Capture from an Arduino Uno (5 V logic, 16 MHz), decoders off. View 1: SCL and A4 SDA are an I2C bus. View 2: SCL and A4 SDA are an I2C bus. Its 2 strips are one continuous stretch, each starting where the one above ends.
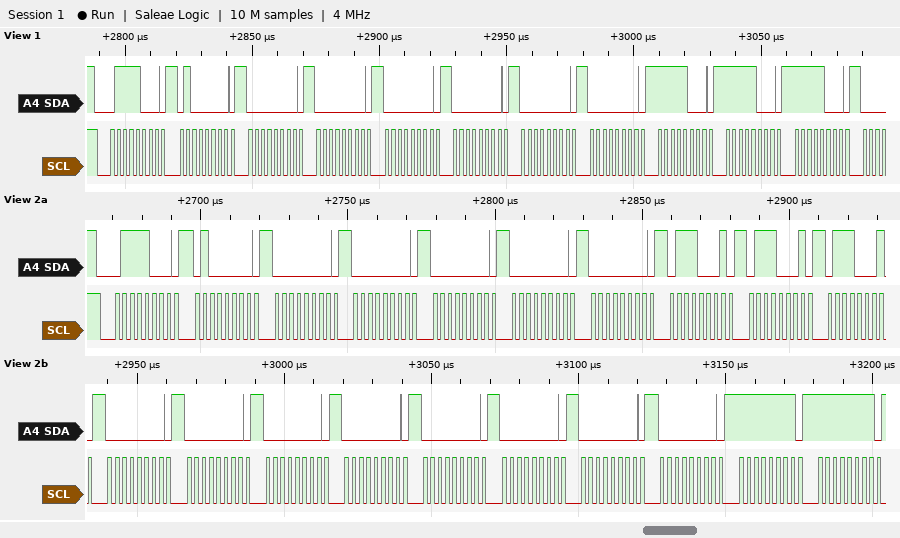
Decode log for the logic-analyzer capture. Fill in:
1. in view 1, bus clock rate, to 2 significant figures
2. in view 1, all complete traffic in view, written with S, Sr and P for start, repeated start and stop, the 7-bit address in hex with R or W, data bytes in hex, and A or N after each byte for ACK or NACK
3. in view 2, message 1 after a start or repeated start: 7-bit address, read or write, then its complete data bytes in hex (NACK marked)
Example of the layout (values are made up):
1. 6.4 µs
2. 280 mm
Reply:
1. 400 kHz
2. S 3CW A 40 A 00 A 00 A 00 A 00 A 00 A 00 A F8 A F8 A F8 A
3. 0x3C write: 40 00 00 00 00 00 71 71 71 00 00 00 00 00 00 00 00 FF FF
